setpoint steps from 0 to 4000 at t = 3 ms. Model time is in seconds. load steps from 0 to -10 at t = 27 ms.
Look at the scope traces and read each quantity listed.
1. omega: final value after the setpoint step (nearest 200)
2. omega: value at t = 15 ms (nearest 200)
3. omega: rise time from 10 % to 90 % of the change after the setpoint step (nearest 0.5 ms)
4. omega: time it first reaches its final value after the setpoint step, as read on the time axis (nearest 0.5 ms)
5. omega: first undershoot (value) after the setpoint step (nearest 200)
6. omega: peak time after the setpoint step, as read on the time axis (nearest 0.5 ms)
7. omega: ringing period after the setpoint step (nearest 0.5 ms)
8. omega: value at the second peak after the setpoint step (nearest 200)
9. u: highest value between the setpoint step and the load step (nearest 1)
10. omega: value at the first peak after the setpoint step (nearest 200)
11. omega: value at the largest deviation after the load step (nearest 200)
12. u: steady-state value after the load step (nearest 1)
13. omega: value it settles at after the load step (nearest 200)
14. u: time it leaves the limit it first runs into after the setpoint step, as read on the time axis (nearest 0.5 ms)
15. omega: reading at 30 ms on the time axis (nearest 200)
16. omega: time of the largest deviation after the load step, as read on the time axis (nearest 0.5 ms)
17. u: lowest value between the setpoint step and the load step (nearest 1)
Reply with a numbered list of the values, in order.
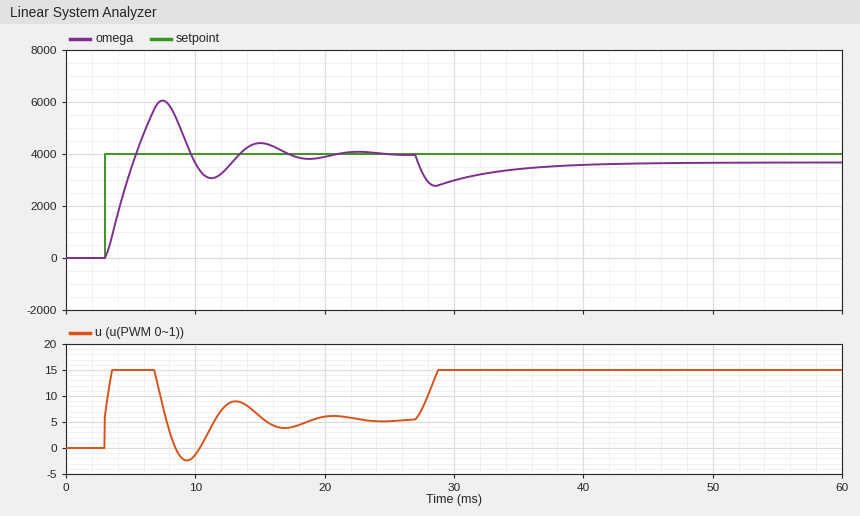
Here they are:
1. 4000
2. 4400
3. 2.0 ms
4. 5.5 ms
5. 3000
6. 7.5 ms
7. 7.5 ms
8. 4400
9. 15
10. 6000
11. 2800
12. 15
13. 3600
14. 7.0 ms
15. 3000
16. 28.5 ms
17. -2
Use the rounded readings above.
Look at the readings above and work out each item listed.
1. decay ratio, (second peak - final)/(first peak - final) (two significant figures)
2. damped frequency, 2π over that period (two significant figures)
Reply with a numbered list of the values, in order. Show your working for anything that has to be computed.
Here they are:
1. (4400 - 4000) / (6000 - 4000) = 0.20
2. 2π / 7.5 = 0.84 rad/ms
